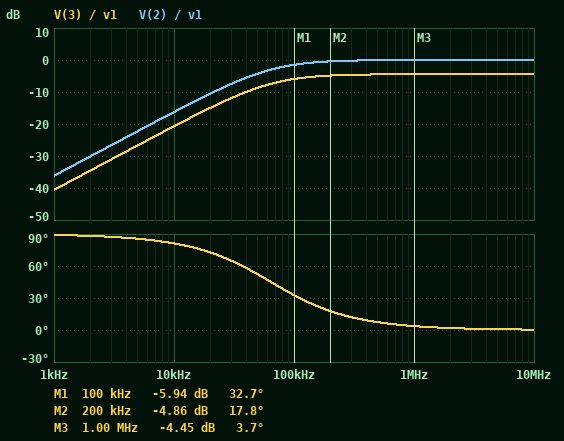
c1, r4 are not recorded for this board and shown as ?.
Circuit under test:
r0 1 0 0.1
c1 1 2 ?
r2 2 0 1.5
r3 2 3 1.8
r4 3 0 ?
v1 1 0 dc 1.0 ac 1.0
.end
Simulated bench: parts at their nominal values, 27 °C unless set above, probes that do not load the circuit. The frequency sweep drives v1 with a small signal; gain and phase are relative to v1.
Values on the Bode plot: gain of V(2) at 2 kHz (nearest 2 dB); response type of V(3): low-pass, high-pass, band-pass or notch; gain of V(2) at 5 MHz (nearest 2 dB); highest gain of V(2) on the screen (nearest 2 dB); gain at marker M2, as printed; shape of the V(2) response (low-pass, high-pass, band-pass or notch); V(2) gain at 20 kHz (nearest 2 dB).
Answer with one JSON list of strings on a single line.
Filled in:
["-30 dB", "high-pass", "0 dB", "0 dB", "-4.86 dB", "high-pass", "-10 dB"]
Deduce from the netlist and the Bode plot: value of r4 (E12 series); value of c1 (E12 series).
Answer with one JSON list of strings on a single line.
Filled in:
["2.7 Ω", "2.2 µF"]
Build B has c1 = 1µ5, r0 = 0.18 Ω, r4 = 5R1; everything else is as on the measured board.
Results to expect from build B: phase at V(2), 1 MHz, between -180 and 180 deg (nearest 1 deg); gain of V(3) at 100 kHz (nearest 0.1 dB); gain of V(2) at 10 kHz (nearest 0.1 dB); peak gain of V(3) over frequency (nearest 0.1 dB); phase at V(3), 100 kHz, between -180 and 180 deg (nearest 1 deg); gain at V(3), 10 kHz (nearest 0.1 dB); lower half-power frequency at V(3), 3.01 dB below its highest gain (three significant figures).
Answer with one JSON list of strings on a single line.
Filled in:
["5 deg", "-5.0 dB", "-18.8 dB", "-2.6 dB", "41 deg", "-21.4 dB", "86.1 kHz"]
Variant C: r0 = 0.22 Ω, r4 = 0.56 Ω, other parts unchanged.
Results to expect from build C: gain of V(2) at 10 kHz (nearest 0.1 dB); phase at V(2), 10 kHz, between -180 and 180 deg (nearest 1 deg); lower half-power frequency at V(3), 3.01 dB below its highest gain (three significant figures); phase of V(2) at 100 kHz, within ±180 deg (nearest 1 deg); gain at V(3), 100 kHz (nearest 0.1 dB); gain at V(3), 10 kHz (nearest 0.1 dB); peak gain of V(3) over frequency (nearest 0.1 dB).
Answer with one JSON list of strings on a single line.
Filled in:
["-18.0 dB", "83 deg", "78.9 kHz", "38 deg", "-14.6 dB", "-30.5 dB", "-12.5 dB"]
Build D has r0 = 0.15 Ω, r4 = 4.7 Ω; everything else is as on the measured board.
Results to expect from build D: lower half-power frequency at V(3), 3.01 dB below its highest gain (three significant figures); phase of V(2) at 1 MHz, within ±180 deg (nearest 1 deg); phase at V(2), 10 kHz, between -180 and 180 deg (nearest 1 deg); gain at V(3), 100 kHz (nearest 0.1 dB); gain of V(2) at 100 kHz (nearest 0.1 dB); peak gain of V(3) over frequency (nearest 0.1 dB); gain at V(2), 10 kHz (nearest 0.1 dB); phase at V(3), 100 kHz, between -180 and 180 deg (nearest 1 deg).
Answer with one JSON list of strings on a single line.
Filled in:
["59.4 kHz", "3 deg", "80 deg", "-4.1 dB", "-1.3 dB", "-2.8 dB", "-15.6 dB", "31 deg"]
